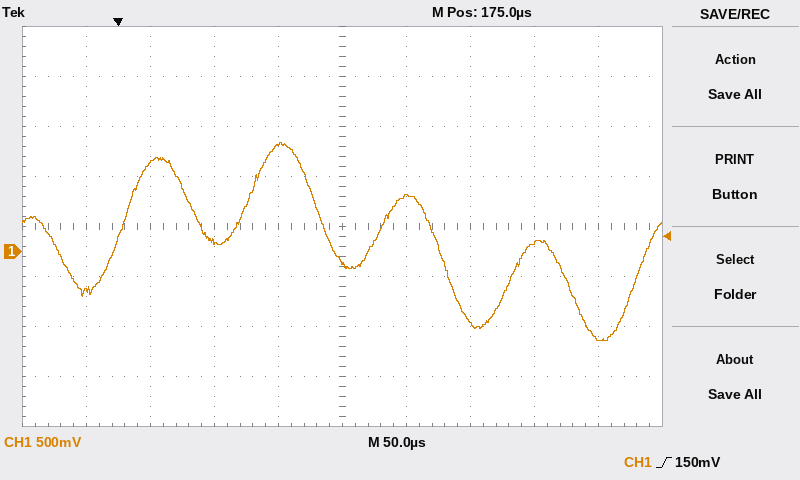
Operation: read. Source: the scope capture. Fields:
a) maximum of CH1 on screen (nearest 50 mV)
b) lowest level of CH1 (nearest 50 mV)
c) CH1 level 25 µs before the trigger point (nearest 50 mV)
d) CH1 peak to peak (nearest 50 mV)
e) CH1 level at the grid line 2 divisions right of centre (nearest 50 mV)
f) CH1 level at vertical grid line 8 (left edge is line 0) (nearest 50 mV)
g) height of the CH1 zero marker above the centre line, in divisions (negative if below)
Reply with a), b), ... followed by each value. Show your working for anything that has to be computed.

a) 1.10 V
b) -900 mV
c) -400 mV
d) 1.10 V − (-900 mV) = 2.00 V
e) -700 mV
f) 100 mV
g) -0.5 div
